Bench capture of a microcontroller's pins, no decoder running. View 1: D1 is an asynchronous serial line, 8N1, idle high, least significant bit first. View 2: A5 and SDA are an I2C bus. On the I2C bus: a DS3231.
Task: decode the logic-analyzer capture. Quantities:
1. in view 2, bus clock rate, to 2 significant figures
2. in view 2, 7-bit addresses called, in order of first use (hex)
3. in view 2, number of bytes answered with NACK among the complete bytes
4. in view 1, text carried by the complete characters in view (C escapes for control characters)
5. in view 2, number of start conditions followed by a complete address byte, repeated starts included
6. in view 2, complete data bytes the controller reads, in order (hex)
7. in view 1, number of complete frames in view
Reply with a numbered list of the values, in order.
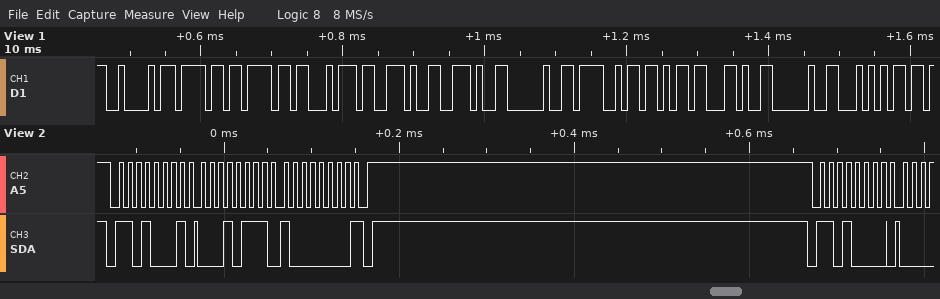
1. 100 kHz
2. 0x68
3. 1
4. "Boot.. Ok, T"
5. 2
6. 17 80
7. 12
